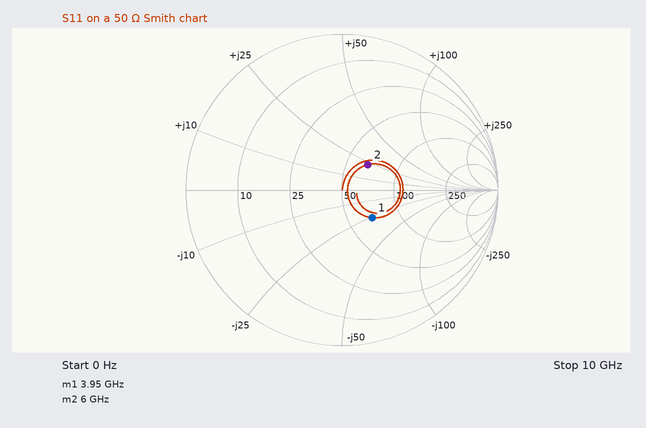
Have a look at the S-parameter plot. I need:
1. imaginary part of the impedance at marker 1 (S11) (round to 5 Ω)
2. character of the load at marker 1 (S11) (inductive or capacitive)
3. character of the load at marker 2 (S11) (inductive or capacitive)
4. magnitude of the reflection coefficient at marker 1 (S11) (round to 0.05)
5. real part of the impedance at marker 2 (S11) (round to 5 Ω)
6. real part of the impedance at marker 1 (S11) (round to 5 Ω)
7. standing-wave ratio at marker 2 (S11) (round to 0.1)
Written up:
-25 Ω
capacitive
inductive
0.25
65 Ω
70 Ω
1.6
